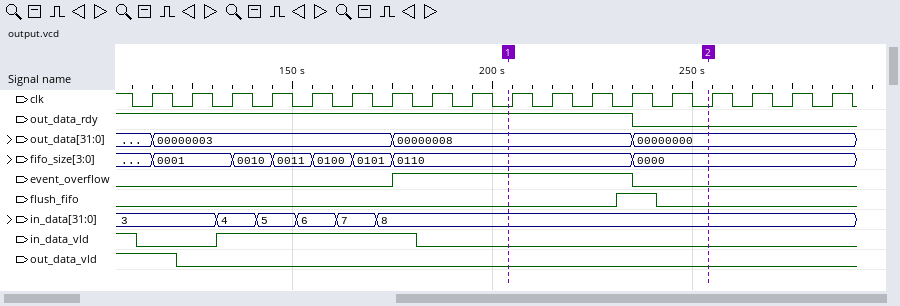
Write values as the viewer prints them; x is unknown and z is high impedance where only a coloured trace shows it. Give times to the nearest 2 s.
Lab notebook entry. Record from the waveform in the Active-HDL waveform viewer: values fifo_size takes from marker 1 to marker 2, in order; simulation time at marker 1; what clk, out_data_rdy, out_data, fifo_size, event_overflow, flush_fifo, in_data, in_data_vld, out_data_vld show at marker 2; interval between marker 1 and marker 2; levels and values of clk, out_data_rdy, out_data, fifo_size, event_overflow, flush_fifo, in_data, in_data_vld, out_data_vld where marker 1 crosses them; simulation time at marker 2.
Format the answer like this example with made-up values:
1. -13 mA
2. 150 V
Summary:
1. 0110, 0000
2. 204 s
3. clk=0, out_data_rdy=0, out_data=00000000, fifo_size=0000, event_overflow=0, flush_fifo=0, in_data=8, in_data_vld=0, out_data_vld=0
4. 50 s
5. clk=0, out_data_rdy=1, out_data=00000008, fifo_size=0110, event_overflow=1, flush_fifo=0, in_data=8, in_data_vld=0, out_data_vld=0
6. 254 s
